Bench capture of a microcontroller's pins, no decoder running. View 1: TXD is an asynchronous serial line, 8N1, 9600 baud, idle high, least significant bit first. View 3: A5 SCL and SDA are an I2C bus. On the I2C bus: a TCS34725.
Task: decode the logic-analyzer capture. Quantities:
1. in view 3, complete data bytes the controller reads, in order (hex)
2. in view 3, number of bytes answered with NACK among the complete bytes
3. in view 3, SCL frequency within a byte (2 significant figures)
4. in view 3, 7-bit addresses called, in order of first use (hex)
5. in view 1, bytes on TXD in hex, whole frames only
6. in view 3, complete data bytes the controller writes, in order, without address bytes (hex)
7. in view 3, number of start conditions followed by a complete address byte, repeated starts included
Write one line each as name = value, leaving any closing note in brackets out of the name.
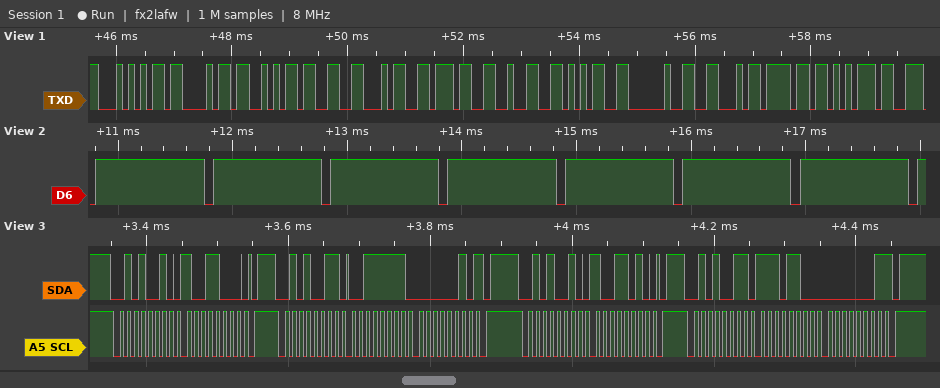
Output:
in view 3, complete data bytes the controller reads, in order = 3F 02 EC 01
in view 3, number of bytes answered with NACK among the complete bytes = 2
in view 3, SCL frequency within a byte = 100 kHz
in view 3, 7-bit addresses called, in order of first use = 0x29
in view 1, bytes on TXD in hex, whole frames only = 54 43 53 33 34 37 32 35 20 46 6F 75
in view 3, complete data bytes the controller writes, in order, without address bytes = 98 9A
in view 3, number of start conditions followed by a complete address byte, repeated starts included = 4
